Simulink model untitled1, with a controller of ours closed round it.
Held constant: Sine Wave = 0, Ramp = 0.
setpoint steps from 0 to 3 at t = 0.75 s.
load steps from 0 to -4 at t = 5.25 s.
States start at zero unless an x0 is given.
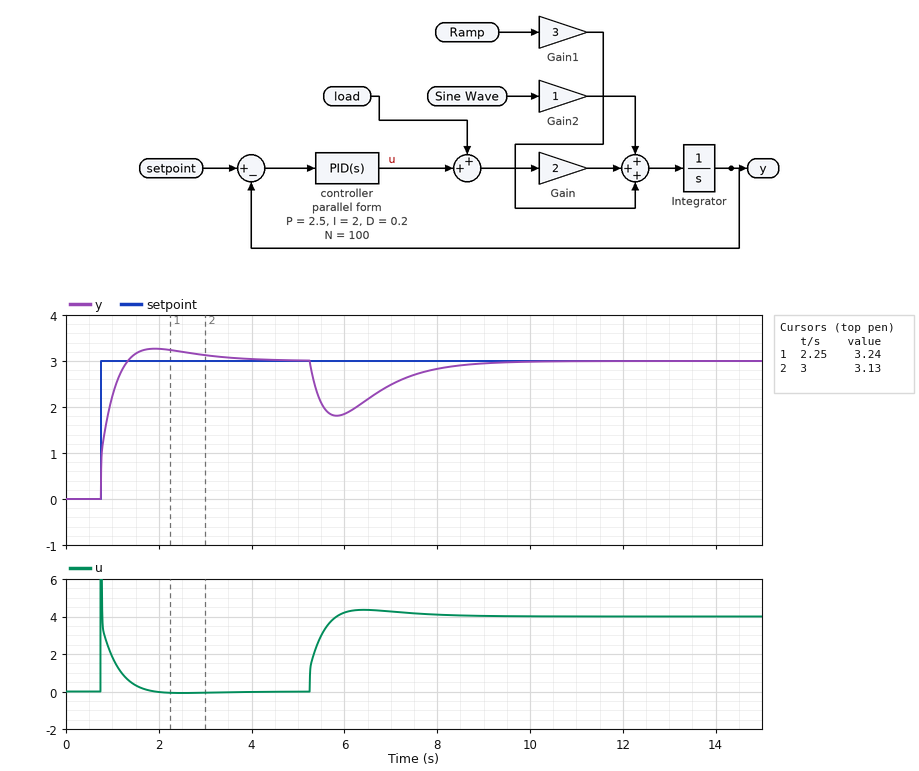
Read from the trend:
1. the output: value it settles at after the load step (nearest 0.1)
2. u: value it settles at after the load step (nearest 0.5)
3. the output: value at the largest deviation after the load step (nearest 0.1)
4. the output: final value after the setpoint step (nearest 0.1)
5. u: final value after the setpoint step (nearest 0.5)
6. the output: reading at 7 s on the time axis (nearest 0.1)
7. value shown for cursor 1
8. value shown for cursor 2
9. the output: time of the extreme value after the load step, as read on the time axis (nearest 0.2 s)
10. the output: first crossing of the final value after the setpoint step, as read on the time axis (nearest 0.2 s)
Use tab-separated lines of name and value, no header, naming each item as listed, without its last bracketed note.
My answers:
the output: value it settles at after the load step	3.0
u: value it settles at after the load step	4.0
the output: value at the largest deviation after the load step	1.8
the output: final value after the setpoint step	3.0
u: final value after the setpoint step	0.0
the output: reading at 7 s on the time axis	2.5
value shown for cursor 1	3.24
value shown for cursor 2	3.13
the output: time of the extreme value after the load step, as read on the time axis	5.8 s
the output: first crossing of the final value after the setpoint step, as read on the time axis	1.4 s
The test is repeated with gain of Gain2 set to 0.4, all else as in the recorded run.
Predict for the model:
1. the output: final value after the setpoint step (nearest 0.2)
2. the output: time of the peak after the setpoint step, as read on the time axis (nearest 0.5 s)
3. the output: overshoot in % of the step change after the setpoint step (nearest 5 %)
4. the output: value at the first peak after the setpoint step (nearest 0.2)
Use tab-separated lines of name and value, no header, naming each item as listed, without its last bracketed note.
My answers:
the output: final value after the setpoint step	3.0
the output: time of the peak after the setpoint step, as read on the time axis	2.0 s
the output: overshoot in % of the step change after the setpoint step	10 %
the output: value at the first peak after the setpoint step	3.2
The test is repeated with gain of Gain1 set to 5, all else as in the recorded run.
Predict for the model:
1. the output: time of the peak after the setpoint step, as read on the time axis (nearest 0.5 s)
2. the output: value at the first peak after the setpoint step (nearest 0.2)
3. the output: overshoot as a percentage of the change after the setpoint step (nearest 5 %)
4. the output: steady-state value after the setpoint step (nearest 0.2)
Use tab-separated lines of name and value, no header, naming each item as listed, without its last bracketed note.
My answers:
the output: time of the peak after the setpoint step, as read on the time axis	2.0 s
the output: value at the first peak after the setpoint step	3.2
the output: overshoot as a percentage of the change after the setpoint step	10 %
the output: steady-state value after the setpoint step	3.0
